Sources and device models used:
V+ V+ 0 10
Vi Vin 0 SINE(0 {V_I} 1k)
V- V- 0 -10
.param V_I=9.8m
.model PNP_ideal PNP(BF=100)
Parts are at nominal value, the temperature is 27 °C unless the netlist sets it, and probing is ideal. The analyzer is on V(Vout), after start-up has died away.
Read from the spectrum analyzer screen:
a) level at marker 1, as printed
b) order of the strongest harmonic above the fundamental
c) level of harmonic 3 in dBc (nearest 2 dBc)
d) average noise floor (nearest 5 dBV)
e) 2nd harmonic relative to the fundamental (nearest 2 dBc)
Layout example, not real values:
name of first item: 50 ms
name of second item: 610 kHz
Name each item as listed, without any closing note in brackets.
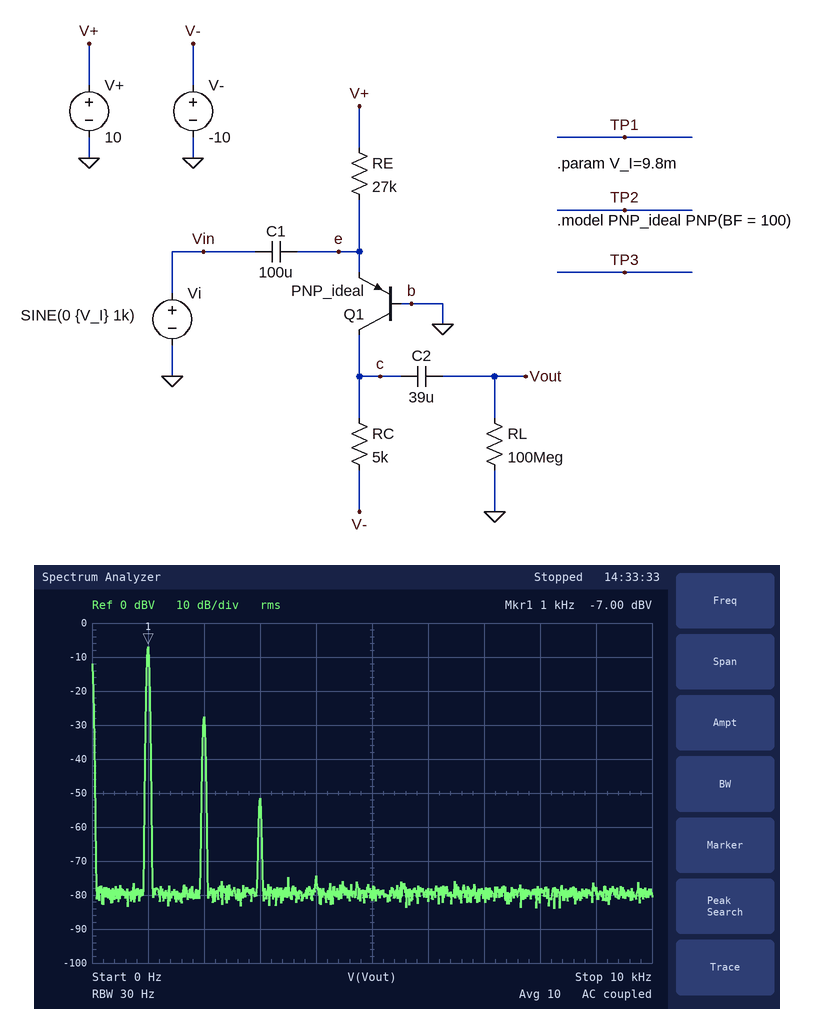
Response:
level at marker 1, as printed: -7.00 dBV
order of the strongest harmonic above the fundamental: 2
level of harmonic 3 in dBc: -44 dBc
average noise floor: -80 dBV
2nd harmonic relative to the fundamental: -20 dBc
